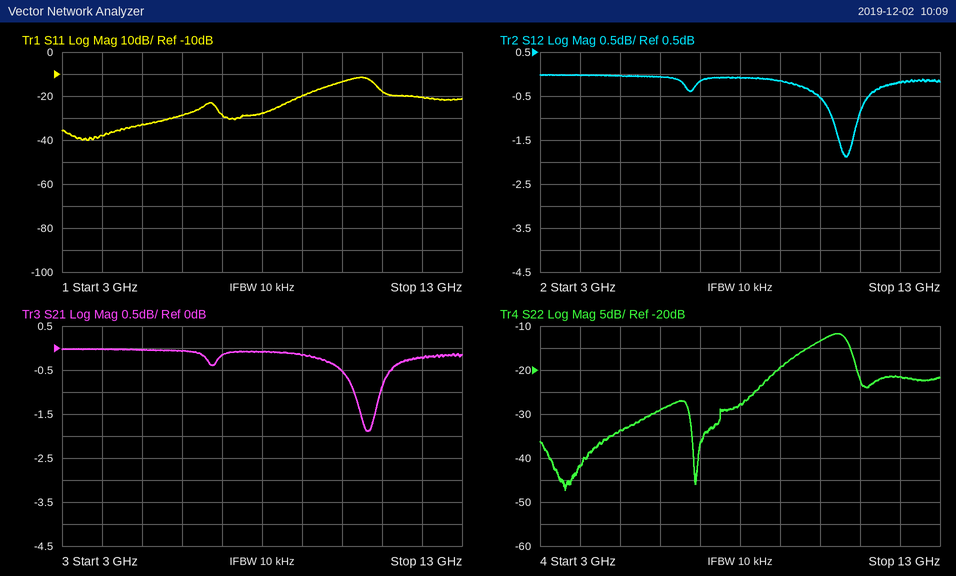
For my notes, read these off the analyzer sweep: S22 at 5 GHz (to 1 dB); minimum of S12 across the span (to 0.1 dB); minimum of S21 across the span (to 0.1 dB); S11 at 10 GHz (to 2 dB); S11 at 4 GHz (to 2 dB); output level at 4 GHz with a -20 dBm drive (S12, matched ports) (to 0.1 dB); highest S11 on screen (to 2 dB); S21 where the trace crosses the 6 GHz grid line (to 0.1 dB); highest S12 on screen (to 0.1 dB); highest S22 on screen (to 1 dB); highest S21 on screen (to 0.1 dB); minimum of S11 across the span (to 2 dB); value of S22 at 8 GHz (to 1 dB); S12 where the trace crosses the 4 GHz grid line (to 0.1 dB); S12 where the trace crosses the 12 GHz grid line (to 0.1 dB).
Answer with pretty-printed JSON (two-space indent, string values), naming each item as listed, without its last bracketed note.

{
  "S22 at 5 GHz": "-34 dB",
  "minimum of S12 across the span": "-1.9 dB",
  "minimum of S21 across the span": "-1.9 dB",
  "S11 at 10 GHz": "-14 dB",
  "S11 at 4 GHz": "-38 dB",
  "output level at 4 GHz with a -20 dBm drive (S12, matched ports)": "-20.0 dBm",
  "highest S11 on screen": "-12 dB",
  "S21 where the trace crosses the 6 GHz grid line": "-0.1 dB",
  "highest S12 on screen": "0.0 dB",
  "highest S22 on screen": "-12 dB",
  "highest S21 on screen": "0.0 dB",
  "minimum of S11 across the span": "-40 dB",
  "value of S22 at 8 GHz": "-28 dB",
  "S12 where the trace crosses the 4 GHz grid line": "0.0 dB",
  "S12 where the trace crosses the 12 GHz grid line": "-0.2 dB"
}
